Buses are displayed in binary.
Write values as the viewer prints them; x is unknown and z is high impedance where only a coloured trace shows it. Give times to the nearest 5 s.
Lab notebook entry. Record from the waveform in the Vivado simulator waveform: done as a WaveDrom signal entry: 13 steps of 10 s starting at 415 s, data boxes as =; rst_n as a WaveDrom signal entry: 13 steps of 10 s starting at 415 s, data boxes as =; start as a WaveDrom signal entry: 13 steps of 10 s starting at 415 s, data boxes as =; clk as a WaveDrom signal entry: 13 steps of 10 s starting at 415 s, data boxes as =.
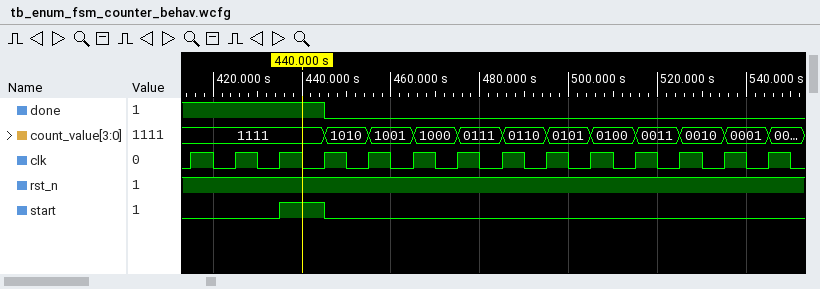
{name: 'done', wave: '1..0.........'}
{name: 'rst_n', wave: '1............'}
{name: 'start', wave: '0.10.........'}
{name: 'clk', wave: 'p............'}
